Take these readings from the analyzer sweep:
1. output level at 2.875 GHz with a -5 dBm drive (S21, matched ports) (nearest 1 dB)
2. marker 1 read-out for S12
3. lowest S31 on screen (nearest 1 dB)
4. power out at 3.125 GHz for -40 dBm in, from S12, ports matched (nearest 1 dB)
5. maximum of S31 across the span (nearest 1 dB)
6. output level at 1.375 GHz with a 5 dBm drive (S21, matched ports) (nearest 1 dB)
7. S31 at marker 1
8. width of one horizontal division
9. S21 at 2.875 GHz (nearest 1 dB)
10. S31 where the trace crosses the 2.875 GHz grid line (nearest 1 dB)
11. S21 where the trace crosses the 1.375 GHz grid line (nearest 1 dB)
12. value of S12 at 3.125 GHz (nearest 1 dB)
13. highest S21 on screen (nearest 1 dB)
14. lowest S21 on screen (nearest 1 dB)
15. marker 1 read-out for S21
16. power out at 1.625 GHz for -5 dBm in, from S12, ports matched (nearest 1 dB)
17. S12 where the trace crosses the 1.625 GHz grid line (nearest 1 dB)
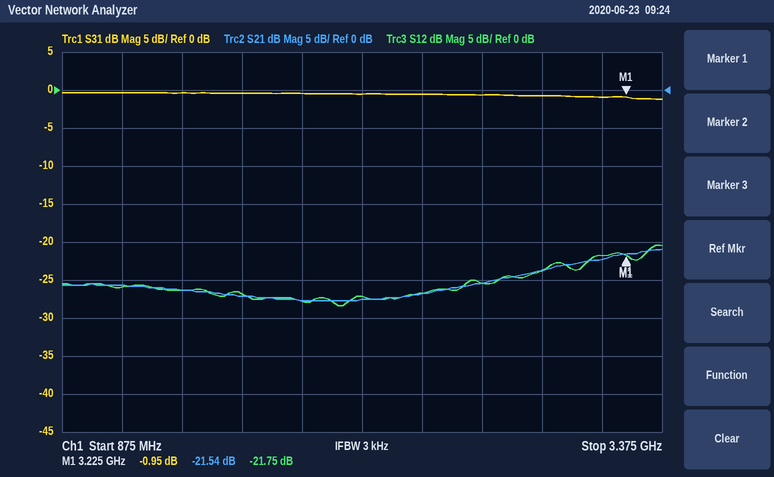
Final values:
-29 dBm
-21.75 dB
-1 dB
-62 dBm
0 dB
-21 dBm
-0.95 dB
250 MHz
-24 dB
-1 dB
-26 dB
-22 dB
-21 dB
-28 dB
-21.54 dB
-32 dBm
-27 dB
